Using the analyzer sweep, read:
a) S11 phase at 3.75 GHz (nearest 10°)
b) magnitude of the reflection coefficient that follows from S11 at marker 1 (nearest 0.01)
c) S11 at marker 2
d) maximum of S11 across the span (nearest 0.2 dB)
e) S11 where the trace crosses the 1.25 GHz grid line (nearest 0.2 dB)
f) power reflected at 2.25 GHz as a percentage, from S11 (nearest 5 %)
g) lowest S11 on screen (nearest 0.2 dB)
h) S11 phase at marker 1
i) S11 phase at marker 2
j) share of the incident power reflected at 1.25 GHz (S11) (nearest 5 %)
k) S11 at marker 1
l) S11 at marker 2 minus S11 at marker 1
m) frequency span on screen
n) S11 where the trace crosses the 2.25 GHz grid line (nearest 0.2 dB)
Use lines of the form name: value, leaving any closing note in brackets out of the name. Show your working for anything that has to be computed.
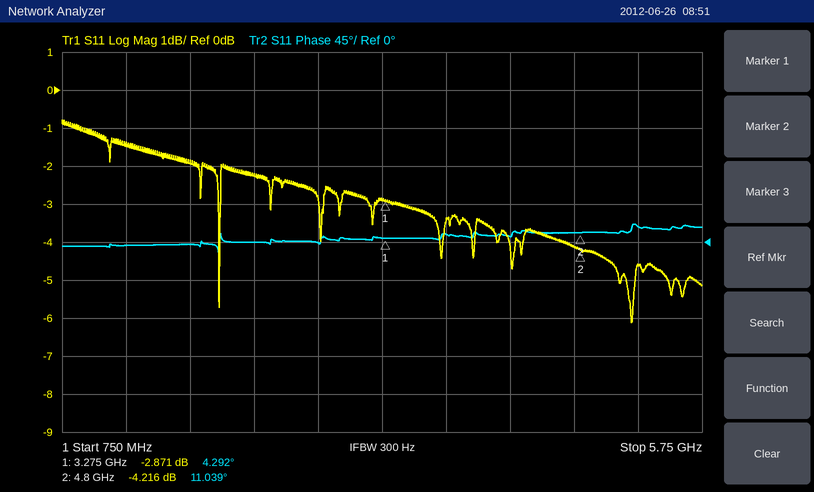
S11 phase at 3.75 GHz: 10°
magnitude of the reflection coefficient that follows from S11 at marker 1: 10^(-2.871/20) ≈ 0.72
S11 at marker 2: -4.216 dB
maximum of S11 across the span: -0.8 dB
S11 where the trace crosses the 1.25 GHz grid line: -1.4 dB
power reflected at 2.25 GHz as a percentage, from S11: 10^(-2.2/10) ≈ 60 %
lowest S11 on screen: -6.2 dB
S11 phase at marker 1: 4.292°
S11 phase at marker 2: 11.039°
share of the incident power reflected at 1.25 GHz (S11): 10^(-1.4/10) ≈ 72.4 %, so 70 % to the nearest 5 %
S11 at marker 1: -2.871 dB
S11 at marker 2 minus S11 at marker 1: -4.216 − (-2.871) = -1.345 dB
frequency span on screen: 5 GHz
S11 where the trace crosses the 2.25 GHz grid line: -2.2 dB
